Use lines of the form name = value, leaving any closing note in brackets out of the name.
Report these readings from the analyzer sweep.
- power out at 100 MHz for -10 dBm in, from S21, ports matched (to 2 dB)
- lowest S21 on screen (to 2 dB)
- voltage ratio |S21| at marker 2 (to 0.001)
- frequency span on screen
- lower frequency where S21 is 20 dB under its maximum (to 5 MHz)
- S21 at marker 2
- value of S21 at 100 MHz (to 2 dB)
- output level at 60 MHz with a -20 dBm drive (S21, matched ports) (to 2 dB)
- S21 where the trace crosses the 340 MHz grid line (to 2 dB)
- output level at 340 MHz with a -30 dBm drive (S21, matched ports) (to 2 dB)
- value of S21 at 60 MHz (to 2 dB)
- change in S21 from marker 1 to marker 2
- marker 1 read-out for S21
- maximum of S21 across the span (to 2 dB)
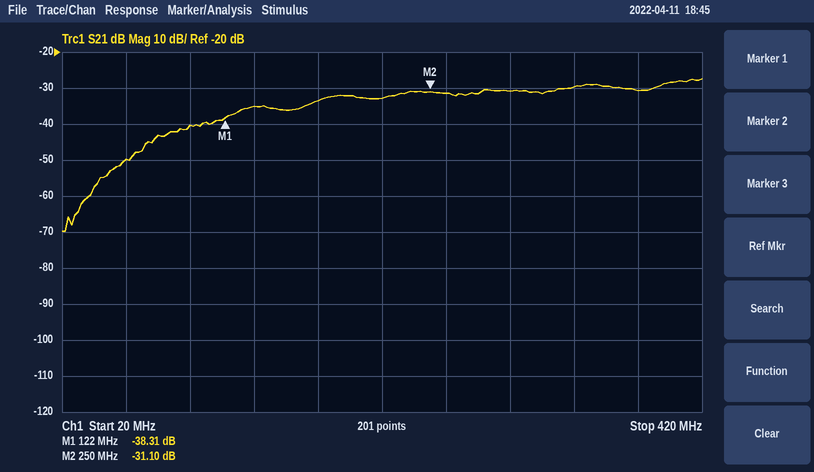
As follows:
power out at 100 MHz for -10 dBm in, from S21, ports matched = -50 dBm
lowest S21 on screen = -70 dB
voltage ratio |S21| at marker 2 = 0.028
frequency span on screen = 400 MHz
lower frequency where S21 is 20 dB under its maximum = 70 MHz
S21 at marker 2 = -31.10 dB
value of S21 at 100 MHz = -40 dB
output level at 60 MHz with a -20 dBm drive (S21, matched ports) = -70 dBm
S21 where the trace crosses the 340 MHz grid line = -30 dB
output level at 340 MHz with a -30 dBm drive (S21, matched ports) = -60 dBm
value of S21 at 60 MHz = -50 dB
change in S21 from marker 1 to marker 2 = 7.21 dB
marker 1 read-out for S21 = -38.31 dB
maximum of S21 across the span = -28 dB
